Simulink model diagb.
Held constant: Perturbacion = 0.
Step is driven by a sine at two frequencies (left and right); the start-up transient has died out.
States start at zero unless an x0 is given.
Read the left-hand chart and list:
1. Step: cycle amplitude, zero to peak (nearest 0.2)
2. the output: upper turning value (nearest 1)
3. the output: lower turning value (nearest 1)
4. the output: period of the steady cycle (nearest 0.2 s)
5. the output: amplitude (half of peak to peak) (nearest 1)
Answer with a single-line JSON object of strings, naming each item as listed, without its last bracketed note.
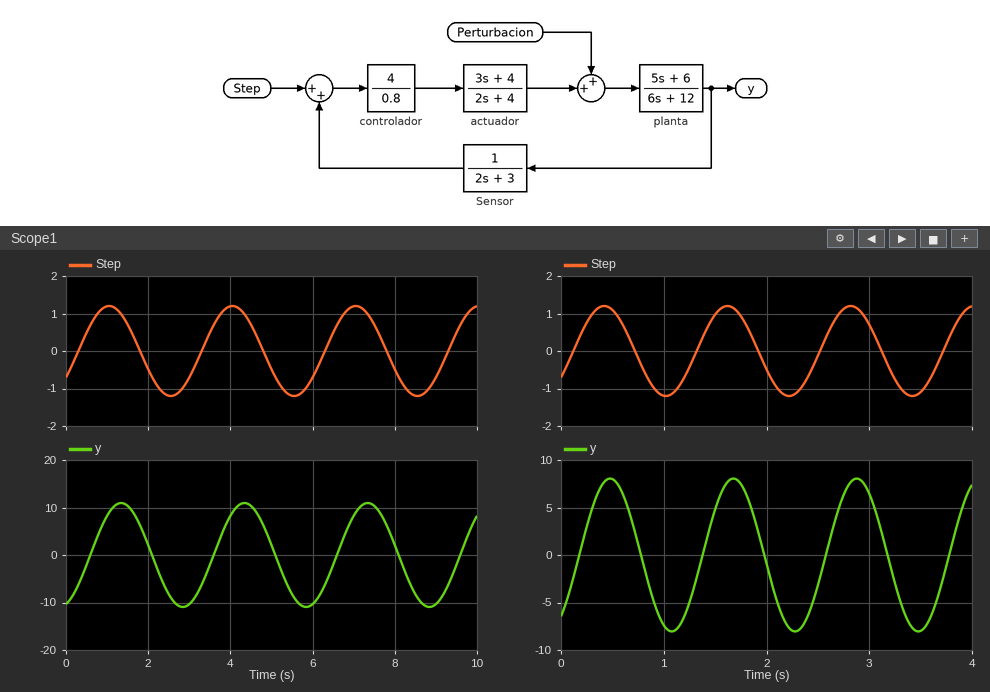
{"Step: cycle amplitude, zero to peak": "1.2", "the output: upper turning value": "11", "the output: lower turning value": "-11", "the output: period of the steady cycle": "3.0 s", "the output: amplitude (half of peak to peak)": "11"}
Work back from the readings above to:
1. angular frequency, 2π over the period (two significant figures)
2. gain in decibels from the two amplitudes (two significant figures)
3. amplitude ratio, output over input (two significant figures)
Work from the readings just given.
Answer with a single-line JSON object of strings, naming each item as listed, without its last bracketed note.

{"angular frequency, 2π over the period": "2.1 rad/s", "gain in decibels from the two amplitudes": "19 dB", "amplitude ratio, output over input": "9.2"}
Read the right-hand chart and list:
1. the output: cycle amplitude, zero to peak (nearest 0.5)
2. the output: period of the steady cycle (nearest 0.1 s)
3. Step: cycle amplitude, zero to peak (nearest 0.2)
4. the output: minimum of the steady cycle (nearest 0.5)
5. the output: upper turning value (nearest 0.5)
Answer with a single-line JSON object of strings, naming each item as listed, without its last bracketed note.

{"the output: cycle amplitude, zero to peak": "8.0", "the output: period of the steady cycle": "1.2 s", "Step: cycle amplitude, zero to peak": "1.2", "the output: minimum of the steady cycle": "-8.0", "the output: upper turning value": "8.0"}
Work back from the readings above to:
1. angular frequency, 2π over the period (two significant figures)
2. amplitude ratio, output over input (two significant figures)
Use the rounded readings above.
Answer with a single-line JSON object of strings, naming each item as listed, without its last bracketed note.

{"angular frequency, 2π over the period": "5.2 rad/s", "amplitude ratio, output over input": "6.7"}
